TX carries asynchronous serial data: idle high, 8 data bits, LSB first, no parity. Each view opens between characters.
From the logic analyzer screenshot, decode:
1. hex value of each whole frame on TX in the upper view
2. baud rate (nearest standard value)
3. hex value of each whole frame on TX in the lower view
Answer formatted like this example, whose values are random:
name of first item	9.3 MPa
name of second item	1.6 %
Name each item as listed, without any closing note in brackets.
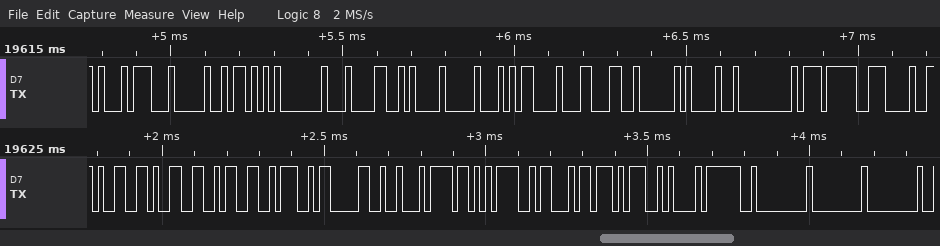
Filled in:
hex value of each whole frame on TX in the upper view	D1, 04, 5A, 01, 84, 0A, 10, 0D, 8C, 02, 21, 00, F7, 0E
baud rate	57600 baud
hex value of each whole frame on TX in the lower view	99, 99, 9A, 3A, 83, 12, 6F, 3D, A3, D7, 0A, 3F, 00, 00, 00
